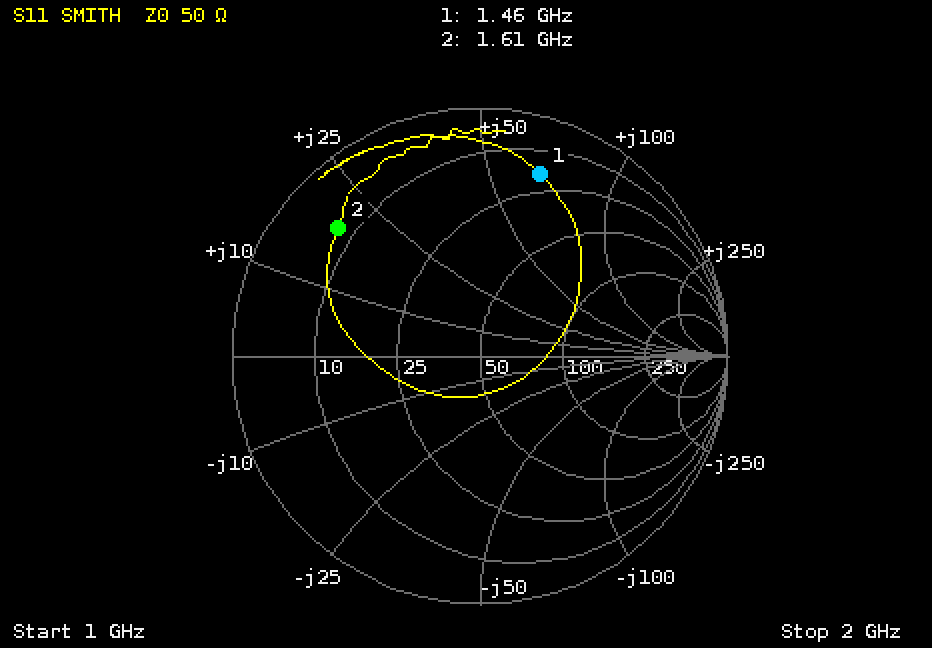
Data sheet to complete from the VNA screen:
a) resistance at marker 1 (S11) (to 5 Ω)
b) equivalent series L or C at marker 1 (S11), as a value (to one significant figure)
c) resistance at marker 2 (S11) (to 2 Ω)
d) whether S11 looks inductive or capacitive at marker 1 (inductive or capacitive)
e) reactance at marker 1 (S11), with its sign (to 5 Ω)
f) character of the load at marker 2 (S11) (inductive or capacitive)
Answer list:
20 Ω
7 nH
8 Ω
inductive
+65 Ω
inductive
